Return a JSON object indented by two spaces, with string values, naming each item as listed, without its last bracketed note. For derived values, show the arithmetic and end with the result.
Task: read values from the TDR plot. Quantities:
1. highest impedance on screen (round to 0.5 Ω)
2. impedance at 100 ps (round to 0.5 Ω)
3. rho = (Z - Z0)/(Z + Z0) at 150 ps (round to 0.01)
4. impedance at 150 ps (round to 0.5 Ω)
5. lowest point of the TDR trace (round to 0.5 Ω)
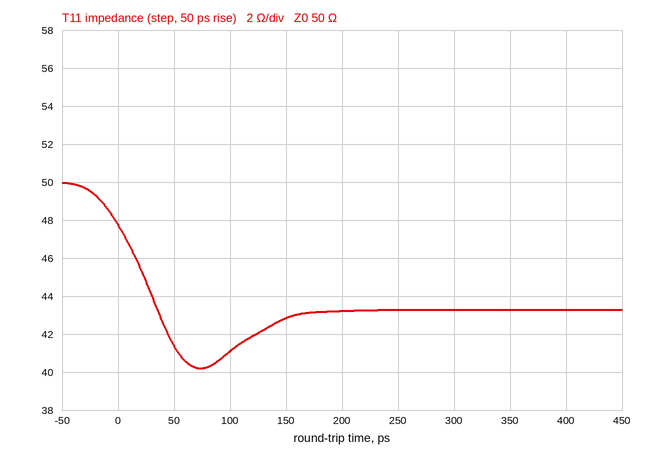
{
  "highest impedance on screen": "50.0 Ω",
  "impedance at 100 ps": "41.0 Ω",
  "rho = (Z - Z0)/(Z + Z0) at 150 ps": "(43 − 50)/(43 + 50) ≈ -0.08",
  "impedance at 150 ps": "43.0 Ω",
  "lowest point of the TDR trace": "40.0 Ω"
}
